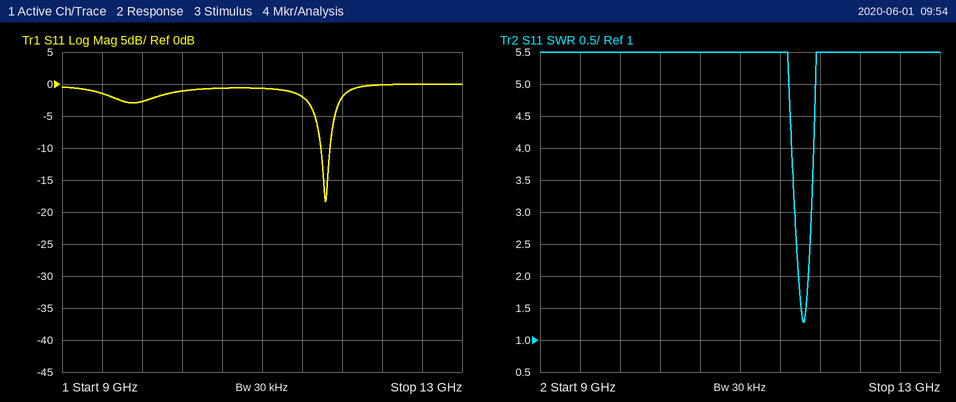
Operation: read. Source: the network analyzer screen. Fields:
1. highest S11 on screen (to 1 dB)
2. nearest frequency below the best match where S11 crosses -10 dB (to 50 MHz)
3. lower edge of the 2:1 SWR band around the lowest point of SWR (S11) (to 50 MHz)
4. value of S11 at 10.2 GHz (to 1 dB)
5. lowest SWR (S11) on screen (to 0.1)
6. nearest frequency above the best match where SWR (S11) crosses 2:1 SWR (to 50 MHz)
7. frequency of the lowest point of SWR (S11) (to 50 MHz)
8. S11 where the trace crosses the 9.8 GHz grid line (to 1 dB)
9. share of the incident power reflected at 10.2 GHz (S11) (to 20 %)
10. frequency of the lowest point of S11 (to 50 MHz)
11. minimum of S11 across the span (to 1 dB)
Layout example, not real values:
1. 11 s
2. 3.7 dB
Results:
1. 0 dB
2. 11.60 GHz
3. 11.60 GHz
4. -1 dB
5. 1.3
6. 11.70 GHz
7. 11.65 GHz
8. -3 dB
9. 80 %
10. 11.65 GHz
11. -18 dB
